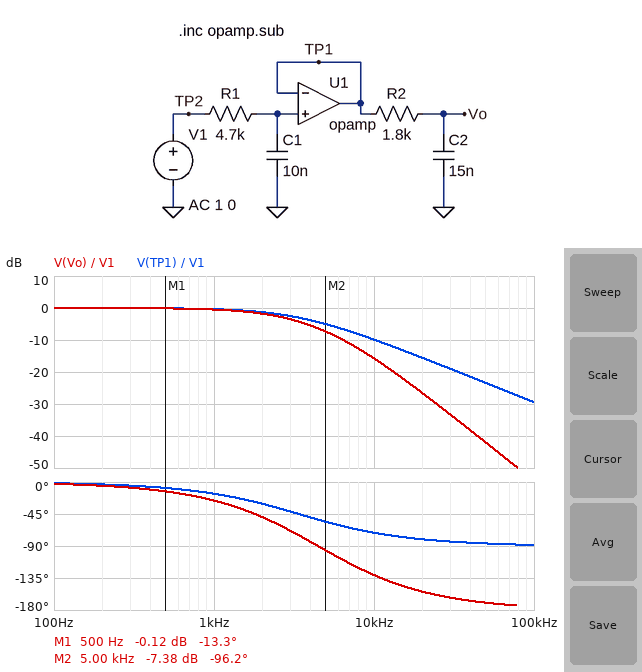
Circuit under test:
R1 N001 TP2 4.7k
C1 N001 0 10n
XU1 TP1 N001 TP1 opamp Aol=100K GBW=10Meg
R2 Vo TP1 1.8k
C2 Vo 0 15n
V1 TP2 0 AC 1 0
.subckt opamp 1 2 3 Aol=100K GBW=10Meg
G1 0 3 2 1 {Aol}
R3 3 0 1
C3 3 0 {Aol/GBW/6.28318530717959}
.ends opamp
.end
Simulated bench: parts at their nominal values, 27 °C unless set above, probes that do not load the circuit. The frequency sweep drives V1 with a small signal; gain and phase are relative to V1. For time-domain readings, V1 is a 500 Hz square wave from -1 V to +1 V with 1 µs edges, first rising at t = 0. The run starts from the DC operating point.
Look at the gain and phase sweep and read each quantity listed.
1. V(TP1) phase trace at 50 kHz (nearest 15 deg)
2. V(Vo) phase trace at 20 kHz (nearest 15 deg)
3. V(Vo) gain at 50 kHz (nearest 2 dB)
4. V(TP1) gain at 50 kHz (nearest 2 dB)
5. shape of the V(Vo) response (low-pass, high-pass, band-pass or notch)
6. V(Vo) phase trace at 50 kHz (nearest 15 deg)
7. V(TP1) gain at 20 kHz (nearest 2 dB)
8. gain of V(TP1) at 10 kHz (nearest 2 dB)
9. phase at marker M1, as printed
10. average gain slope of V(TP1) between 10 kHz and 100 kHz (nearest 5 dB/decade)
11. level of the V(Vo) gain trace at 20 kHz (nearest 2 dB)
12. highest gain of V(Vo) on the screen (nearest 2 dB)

-90 deg
-150 deg
-42 dB
-24 dB
low-pass
-165 deg
-16 dB
-10 dB
-13.3 deg
-20 dB/decade
-26 dB
0 dB
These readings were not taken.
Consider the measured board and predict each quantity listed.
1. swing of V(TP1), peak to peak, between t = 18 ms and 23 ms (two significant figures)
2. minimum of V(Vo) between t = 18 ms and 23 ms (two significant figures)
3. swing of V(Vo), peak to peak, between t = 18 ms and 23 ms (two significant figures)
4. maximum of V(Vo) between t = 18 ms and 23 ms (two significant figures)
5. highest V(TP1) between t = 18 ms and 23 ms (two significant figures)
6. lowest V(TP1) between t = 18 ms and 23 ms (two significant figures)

2.0 V
-1.0 V
2.0 V
1.0 V
1.0 V
-1.0 V
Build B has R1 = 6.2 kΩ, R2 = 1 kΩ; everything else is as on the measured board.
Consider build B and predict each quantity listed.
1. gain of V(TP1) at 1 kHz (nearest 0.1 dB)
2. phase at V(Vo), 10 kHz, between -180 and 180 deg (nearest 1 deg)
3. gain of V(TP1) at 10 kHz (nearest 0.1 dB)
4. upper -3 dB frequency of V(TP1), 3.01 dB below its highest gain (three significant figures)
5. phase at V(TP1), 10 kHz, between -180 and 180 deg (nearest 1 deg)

-0.6 dB
-119 deg
-12.1 dB
2.57 kHz
-76 deg
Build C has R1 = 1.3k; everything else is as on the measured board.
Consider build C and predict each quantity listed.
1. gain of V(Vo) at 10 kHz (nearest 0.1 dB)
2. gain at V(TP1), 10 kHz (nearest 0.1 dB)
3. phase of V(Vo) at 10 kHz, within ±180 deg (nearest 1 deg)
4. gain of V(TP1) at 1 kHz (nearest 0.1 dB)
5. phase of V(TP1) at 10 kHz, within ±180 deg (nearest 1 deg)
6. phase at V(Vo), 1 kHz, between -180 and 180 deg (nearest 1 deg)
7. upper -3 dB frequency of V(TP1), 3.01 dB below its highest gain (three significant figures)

-8.1 dB
-2.2 dB
-99 deg
0 dB
-39 deg
-14 deg
12.2 kHz
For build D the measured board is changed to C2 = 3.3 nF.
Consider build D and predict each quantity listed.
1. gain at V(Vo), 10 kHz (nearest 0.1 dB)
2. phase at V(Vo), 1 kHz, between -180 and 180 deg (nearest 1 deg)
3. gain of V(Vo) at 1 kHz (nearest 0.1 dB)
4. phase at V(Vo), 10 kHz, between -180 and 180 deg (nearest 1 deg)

-10.4 dB
-19 deg
-0.4 dB
-92 deg
